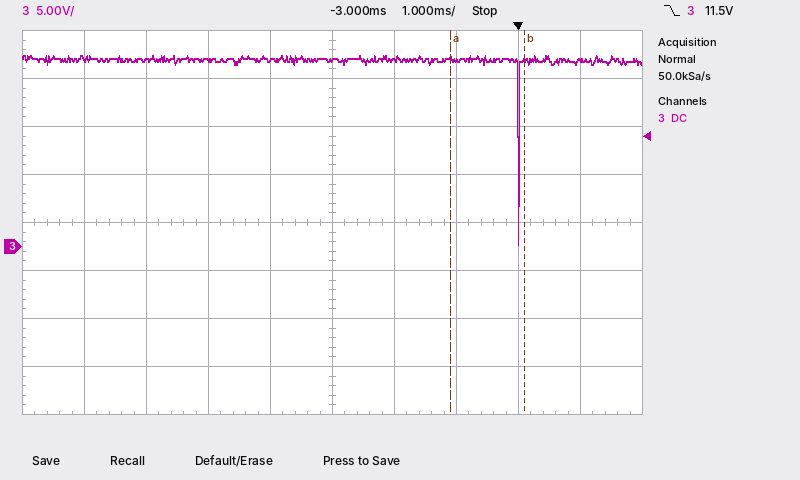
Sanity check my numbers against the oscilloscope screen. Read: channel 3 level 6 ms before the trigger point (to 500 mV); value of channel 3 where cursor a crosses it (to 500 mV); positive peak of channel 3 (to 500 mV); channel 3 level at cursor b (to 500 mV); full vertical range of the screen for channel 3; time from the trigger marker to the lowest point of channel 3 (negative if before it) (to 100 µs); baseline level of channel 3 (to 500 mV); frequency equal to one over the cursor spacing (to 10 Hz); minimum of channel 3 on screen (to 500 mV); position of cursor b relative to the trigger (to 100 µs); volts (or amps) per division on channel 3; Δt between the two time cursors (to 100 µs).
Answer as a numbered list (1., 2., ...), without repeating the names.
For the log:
1. 19.5 V
2. 19.5 V
3. 20.0 V
4. 19.5 V
5. 40 V
6. 0.0 ms
7. 19.5 V
8. 830 Hz
9. 0.0 V
10. +100 µs
11. 5 V
12. 1.2 ms
